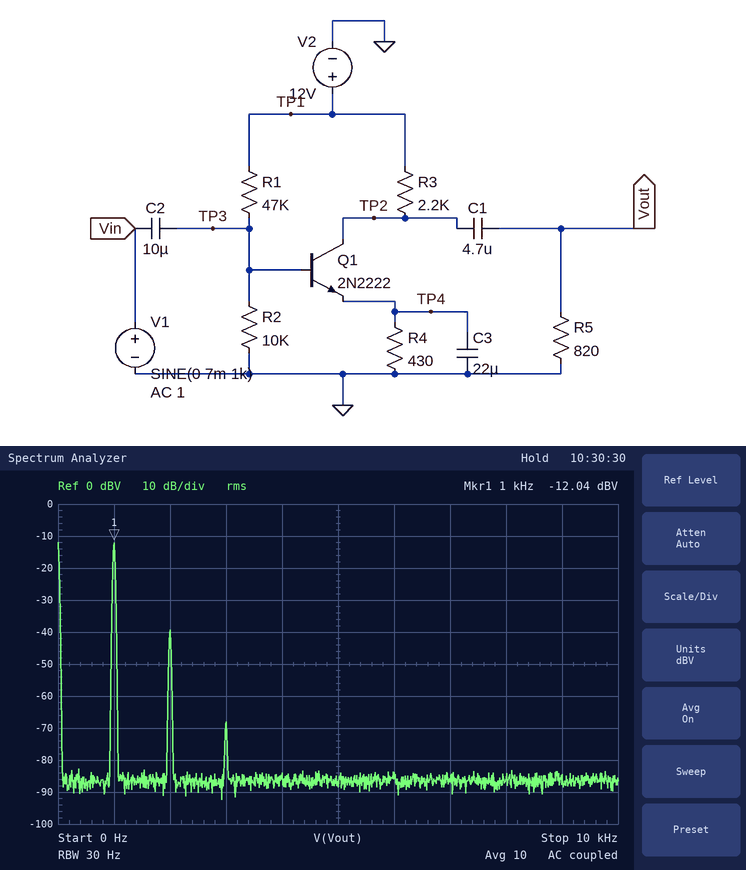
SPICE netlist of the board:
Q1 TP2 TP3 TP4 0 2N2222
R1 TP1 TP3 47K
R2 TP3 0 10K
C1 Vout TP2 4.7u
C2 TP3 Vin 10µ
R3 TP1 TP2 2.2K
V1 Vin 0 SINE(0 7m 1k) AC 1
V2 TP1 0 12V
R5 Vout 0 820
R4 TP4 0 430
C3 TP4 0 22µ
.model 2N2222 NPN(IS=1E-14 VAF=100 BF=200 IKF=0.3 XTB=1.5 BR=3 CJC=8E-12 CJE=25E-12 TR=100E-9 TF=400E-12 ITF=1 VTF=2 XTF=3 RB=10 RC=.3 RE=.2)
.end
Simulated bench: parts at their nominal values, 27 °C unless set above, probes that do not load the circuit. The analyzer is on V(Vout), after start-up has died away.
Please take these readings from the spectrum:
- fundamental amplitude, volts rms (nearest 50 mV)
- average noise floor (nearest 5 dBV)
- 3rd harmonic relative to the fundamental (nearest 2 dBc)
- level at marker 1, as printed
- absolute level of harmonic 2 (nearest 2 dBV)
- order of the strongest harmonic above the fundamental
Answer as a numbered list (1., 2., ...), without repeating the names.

1. 250 mV
2. -85 dBV
3. -56 dBc
4. -12.04 dBV
5. -40 dBV
6. 2
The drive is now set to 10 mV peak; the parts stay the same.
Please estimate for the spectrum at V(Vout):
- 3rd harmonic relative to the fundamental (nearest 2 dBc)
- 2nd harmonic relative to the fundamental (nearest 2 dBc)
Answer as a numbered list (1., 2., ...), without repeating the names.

1. -50 dBc
2. -24 dBc
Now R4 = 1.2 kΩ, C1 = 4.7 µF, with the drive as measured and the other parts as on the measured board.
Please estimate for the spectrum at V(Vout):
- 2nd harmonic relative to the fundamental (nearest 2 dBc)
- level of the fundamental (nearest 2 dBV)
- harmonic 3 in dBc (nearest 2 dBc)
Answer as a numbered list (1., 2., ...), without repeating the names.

1. -24 dBc
2. -18 dBV
3. -52 dBc
